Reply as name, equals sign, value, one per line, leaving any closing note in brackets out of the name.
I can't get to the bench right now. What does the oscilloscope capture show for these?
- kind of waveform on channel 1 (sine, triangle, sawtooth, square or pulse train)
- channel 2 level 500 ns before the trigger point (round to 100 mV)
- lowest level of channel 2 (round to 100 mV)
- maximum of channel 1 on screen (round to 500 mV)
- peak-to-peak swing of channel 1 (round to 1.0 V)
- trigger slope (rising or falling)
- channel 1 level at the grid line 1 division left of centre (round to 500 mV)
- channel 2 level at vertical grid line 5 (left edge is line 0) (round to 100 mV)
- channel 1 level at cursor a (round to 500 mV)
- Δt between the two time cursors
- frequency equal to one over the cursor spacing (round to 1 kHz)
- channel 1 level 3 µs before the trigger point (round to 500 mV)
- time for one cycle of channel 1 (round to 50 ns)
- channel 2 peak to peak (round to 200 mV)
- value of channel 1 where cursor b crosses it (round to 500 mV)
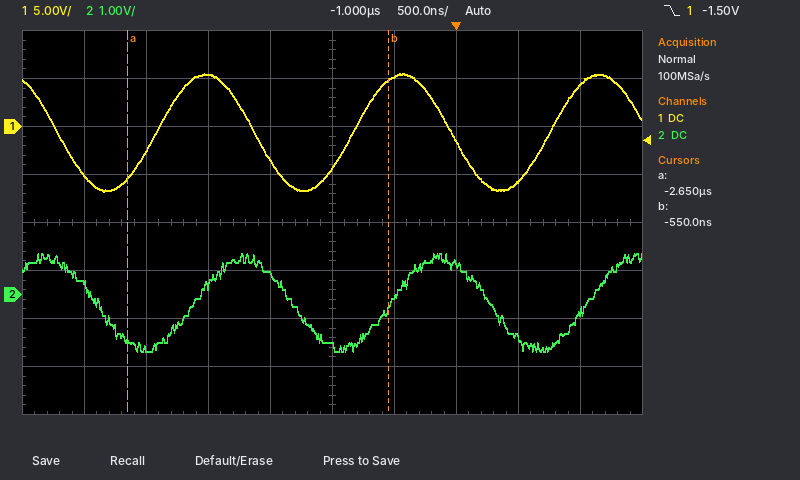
kind of waveform on channel 1 = sine
channel 2 level 500 ns before the trigger point = -100 mV
lowest level of channel 2 = -1.2 V
maximum of channel 1 on screen = 5.5 V
peak-to-peak swing of channel 1 = 12.0 V
trigger slope = falling
channel 1 level at the grid line 1 division left of centre = -3.5 V
channel 2 level at vertical grid line 5 (left edge is line 0) = -1.1 V
channel 1 level at cursor a = -5.5 V
Δt between the two time cursors = 2.10 µs
frequency equal to one over the cursor spacing = 476 kHz
channel 1 level 3 µs before the trigger point = -5.0 V
time for one cycle of channel 1 = 1.60 µs
channel 2 peak to peak = 2.0 V
value of channel 1 where cursor b crosses it = 5.0 V
